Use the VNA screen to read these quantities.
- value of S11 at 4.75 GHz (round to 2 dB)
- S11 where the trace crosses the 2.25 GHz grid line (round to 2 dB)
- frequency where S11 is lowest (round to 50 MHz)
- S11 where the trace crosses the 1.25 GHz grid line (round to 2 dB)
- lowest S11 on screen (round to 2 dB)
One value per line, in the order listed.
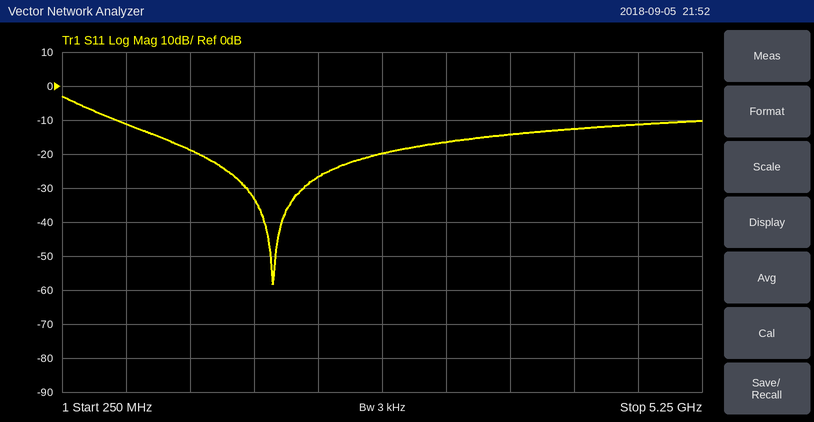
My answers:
-12 dB
-26 dB
1.90 GHz
-18 dB
-58 dB
